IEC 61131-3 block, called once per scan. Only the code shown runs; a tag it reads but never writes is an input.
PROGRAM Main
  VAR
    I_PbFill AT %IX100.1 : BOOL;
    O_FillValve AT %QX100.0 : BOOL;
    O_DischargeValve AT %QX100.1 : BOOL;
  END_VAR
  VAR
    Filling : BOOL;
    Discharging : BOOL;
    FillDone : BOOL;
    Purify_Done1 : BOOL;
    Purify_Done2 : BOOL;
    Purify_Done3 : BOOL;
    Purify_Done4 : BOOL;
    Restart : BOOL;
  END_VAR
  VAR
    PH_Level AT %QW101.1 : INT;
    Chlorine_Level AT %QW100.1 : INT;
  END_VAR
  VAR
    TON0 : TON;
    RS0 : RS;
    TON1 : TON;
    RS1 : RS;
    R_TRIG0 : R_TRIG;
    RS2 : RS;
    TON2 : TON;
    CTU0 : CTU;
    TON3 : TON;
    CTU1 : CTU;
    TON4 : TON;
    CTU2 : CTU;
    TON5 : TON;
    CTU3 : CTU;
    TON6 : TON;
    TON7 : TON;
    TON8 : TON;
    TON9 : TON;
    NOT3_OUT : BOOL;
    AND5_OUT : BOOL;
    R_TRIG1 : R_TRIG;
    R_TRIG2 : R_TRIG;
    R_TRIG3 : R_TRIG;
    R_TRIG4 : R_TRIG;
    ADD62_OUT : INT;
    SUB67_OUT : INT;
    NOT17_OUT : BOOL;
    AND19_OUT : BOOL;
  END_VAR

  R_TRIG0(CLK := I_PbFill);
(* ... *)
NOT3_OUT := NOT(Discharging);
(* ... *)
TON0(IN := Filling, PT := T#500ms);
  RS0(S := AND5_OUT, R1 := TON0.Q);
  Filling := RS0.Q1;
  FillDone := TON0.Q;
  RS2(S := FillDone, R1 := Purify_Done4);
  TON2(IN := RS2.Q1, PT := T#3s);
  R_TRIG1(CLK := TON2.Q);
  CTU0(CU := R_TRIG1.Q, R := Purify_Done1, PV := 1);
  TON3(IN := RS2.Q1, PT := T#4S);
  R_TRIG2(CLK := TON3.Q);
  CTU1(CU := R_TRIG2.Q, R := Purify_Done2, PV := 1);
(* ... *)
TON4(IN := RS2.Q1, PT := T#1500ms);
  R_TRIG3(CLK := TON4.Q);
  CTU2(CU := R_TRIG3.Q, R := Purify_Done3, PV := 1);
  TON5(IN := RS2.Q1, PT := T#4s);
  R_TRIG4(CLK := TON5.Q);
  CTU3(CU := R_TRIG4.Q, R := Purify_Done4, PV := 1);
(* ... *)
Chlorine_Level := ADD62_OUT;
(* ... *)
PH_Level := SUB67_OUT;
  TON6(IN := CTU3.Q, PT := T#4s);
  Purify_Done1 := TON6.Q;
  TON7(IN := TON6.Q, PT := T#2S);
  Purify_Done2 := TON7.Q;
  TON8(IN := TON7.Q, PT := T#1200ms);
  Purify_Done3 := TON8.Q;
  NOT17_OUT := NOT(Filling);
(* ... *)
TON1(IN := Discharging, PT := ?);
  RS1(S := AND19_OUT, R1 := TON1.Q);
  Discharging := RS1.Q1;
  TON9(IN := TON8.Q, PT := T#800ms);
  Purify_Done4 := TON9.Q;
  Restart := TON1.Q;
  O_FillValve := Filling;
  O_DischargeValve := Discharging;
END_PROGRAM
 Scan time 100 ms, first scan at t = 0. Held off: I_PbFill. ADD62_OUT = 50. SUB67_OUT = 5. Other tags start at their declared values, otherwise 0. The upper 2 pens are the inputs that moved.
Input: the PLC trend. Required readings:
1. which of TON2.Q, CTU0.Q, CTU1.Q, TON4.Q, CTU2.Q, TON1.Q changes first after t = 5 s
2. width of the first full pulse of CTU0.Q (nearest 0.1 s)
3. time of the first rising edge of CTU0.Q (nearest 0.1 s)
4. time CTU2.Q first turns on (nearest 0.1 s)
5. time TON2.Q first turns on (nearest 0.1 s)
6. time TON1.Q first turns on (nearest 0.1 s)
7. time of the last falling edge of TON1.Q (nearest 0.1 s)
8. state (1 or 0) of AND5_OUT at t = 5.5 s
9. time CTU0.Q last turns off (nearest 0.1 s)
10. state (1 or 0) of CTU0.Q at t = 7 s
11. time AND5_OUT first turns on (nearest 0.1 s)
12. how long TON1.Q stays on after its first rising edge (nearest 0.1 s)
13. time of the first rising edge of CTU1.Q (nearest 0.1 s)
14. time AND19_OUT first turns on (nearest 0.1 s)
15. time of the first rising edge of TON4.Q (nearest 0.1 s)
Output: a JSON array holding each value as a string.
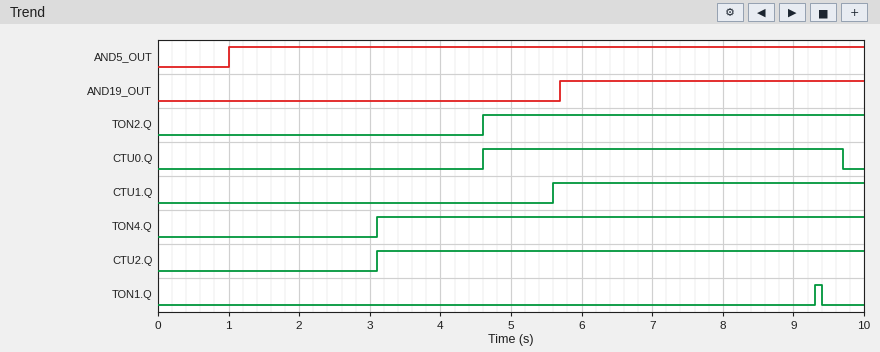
["CTU1.Q", "5.1 s", "4.6 s", "3.1 s", "4.6 s", "9.3 s", "9.4 s", "1", "9.7 s", "1", "1.0 s", "0.1 s", "5.6 s", "5.7 s", "3.1 s"]
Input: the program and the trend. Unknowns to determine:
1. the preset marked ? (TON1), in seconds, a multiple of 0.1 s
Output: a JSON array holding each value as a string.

["3.5 s"]
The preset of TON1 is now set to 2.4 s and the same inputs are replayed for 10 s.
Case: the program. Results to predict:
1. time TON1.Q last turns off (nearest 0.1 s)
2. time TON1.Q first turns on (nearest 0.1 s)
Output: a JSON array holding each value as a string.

["8.3 s", "8.2 s"]
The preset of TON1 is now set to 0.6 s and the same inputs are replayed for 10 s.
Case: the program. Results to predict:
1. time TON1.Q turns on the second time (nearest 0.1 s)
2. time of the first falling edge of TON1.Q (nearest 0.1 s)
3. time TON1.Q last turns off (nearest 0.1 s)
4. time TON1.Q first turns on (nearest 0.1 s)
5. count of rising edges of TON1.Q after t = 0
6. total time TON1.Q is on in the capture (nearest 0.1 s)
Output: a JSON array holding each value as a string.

["7.2 s", "6.5 s", "9.7 s", "6.4 s", "5", "0.5 s"]
